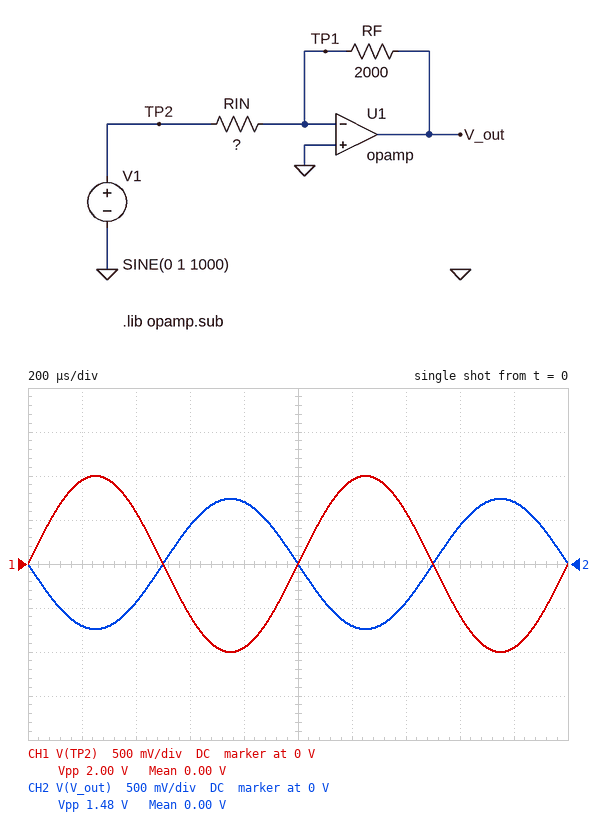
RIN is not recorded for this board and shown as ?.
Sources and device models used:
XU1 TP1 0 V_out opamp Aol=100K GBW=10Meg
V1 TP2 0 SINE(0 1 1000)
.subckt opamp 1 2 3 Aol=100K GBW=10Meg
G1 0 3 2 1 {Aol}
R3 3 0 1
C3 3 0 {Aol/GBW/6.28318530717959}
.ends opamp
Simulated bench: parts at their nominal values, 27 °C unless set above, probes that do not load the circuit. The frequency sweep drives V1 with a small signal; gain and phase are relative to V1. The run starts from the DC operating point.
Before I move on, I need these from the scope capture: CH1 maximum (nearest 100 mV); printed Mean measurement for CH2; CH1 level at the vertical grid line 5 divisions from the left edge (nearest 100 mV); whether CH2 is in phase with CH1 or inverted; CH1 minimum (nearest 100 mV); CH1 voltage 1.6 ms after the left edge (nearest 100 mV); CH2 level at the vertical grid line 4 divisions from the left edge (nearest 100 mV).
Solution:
1.0 V
0.00 V
0 V
inverted
-1.0 V
-600 mV
700 mV
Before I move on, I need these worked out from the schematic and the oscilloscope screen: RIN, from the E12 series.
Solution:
2.7 kΩ
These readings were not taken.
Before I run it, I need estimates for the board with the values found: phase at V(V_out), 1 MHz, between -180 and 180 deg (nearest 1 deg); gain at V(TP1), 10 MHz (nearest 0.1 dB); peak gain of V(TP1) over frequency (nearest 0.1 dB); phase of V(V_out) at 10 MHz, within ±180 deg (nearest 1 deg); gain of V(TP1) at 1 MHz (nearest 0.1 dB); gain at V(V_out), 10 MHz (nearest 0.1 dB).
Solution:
170 deg
-8.7 dB
-7.4 dB
120 deg
-22.7 dB
-8.7 dB
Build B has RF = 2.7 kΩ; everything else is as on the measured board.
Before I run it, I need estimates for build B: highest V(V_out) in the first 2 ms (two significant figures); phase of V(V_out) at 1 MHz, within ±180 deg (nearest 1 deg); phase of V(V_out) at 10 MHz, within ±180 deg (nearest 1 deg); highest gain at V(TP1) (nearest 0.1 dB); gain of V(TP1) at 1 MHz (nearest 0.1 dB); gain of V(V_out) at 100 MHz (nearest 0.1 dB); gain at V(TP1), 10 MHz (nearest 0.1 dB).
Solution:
1.0 V
169 deg
117 deg
-6.0 dB
-20.2 dB
-26.0 dB
-7.0 dB
